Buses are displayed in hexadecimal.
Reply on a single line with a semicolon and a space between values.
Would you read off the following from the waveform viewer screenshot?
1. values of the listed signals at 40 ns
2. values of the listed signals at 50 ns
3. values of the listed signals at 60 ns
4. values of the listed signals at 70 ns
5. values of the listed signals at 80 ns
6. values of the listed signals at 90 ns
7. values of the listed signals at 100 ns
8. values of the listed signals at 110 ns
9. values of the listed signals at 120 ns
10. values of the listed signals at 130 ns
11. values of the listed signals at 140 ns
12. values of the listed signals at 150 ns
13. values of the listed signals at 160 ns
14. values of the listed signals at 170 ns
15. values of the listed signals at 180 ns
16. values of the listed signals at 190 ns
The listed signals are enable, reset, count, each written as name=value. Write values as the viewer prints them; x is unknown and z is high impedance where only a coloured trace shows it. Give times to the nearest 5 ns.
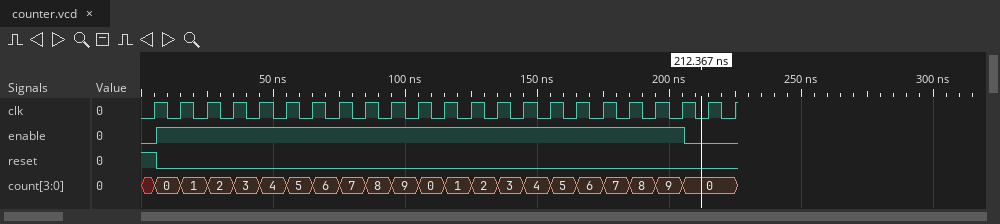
enable=1, reset=0, count=3; enable=1, reset=0, count=4; enable=1, reset=0, count=5; enable=1, reset=0, count=6; enable=1, reset=0, count=7; enable=1, reset=0, count=8; enable=1, reset=0, count=9; enable=1, reset=0, count=0; enable=1, reset=0, count=1; enable=1, reset=0, count=2; enable=1, reset=0, count=3; enable=1, reset=0, count=4; enable=1, reset=0, count=5; enable=1, reset=0, count=6; enable=1, reset=0, count=7; enable=1, reset=0, count=8
